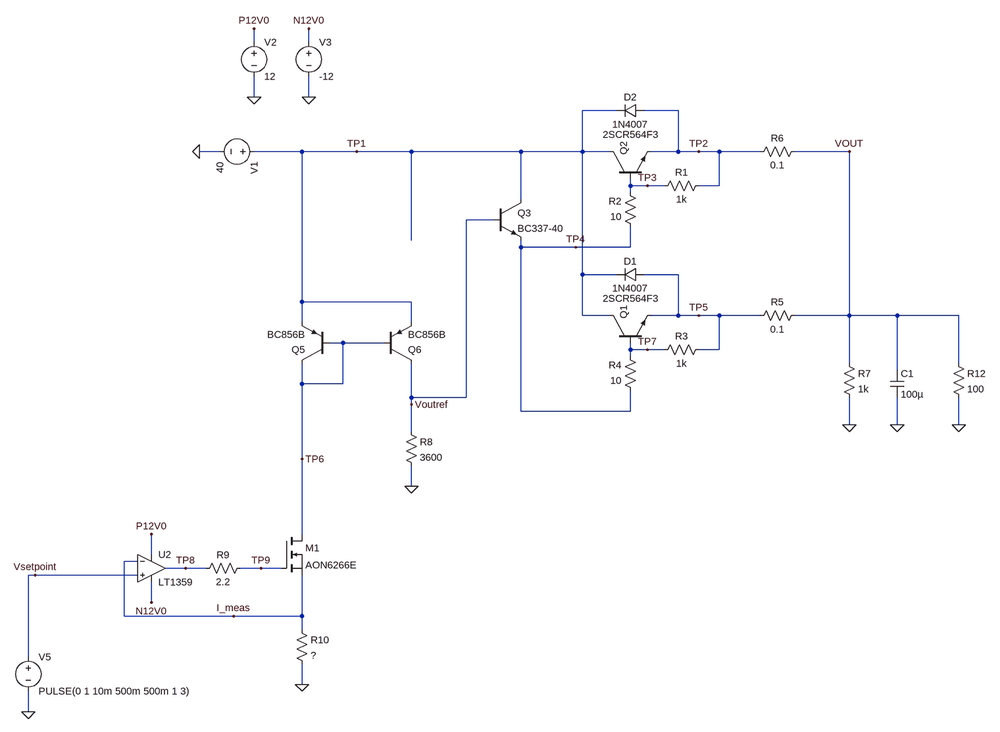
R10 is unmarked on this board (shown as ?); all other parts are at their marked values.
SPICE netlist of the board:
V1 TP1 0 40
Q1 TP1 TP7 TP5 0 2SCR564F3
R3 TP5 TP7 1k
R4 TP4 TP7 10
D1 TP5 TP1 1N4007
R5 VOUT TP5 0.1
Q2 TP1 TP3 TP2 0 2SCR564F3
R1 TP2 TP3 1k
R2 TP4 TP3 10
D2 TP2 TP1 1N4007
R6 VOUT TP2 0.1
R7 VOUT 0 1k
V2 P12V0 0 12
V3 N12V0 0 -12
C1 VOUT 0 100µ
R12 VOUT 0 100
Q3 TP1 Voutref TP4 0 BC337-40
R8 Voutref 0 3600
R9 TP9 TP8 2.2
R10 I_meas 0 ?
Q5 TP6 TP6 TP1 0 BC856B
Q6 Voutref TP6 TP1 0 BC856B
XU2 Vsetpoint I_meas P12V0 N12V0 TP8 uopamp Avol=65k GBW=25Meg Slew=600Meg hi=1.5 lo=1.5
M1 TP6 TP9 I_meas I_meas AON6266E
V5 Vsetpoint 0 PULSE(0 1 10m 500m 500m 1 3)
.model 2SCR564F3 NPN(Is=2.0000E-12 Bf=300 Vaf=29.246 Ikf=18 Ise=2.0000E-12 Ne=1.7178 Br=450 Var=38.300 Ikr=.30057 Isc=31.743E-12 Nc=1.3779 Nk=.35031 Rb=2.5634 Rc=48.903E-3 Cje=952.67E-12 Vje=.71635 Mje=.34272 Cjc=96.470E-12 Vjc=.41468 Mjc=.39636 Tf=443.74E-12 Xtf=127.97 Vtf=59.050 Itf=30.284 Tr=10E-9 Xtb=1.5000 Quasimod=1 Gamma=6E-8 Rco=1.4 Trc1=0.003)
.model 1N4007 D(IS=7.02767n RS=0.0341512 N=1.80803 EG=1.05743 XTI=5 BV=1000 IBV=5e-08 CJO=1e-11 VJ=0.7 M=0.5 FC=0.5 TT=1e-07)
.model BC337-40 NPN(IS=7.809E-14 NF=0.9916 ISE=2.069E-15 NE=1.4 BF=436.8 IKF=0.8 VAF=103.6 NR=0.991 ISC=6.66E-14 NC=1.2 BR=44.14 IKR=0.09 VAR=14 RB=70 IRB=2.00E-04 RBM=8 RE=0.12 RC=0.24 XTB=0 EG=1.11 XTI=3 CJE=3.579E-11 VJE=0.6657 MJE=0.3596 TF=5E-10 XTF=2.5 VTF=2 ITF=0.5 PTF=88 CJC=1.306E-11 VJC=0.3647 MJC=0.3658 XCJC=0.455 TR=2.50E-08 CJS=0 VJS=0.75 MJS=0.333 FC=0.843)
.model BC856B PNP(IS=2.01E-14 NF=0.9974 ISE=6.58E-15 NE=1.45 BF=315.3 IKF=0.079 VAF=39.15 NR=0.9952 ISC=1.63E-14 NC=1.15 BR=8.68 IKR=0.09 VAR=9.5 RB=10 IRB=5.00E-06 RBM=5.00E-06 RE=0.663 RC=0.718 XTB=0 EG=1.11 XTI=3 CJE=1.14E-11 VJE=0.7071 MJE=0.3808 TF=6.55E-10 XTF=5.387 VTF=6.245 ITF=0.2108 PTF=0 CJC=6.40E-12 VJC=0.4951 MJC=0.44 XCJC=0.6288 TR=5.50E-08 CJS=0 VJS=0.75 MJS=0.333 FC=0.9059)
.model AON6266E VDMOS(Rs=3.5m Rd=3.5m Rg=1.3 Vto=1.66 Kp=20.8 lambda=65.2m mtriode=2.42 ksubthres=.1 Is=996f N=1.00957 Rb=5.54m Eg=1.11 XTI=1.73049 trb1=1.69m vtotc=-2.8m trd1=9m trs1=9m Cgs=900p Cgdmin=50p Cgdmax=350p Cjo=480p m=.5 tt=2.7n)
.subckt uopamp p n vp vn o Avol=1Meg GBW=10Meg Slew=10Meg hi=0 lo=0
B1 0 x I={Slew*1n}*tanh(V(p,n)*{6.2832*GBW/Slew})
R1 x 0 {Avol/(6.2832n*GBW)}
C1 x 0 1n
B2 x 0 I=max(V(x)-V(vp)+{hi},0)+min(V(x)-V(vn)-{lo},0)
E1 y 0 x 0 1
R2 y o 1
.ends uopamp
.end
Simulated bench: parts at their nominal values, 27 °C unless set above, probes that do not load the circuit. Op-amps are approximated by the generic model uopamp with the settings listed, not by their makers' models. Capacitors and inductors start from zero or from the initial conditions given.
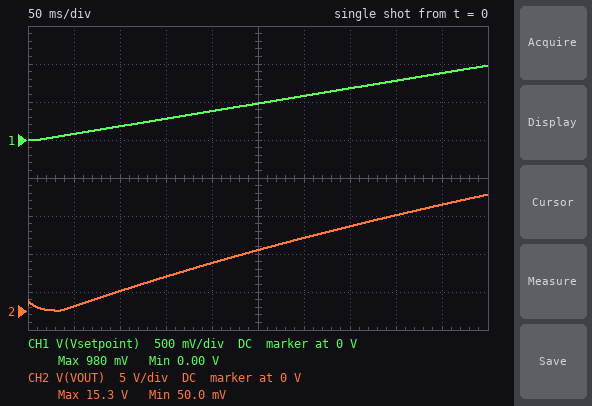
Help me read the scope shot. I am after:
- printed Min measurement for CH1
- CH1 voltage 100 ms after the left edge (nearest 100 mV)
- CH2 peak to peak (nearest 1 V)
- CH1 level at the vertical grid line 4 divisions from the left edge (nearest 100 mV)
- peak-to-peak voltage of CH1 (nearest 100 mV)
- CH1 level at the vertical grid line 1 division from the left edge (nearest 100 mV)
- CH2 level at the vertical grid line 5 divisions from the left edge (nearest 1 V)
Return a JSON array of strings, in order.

["0.00 V", "200 mV", "15 V", "400 mV", "1.0 V", "100 mV", "8 V"]
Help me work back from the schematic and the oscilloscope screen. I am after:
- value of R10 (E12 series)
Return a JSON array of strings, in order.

["330 Ω"]
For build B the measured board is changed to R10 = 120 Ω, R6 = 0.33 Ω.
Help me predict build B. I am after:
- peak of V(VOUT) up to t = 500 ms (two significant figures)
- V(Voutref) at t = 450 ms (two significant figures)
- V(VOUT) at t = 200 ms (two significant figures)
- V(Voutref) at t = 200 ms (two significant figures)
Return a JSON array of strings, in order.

["32 V", "31 V", "16 V", "17 V"]
